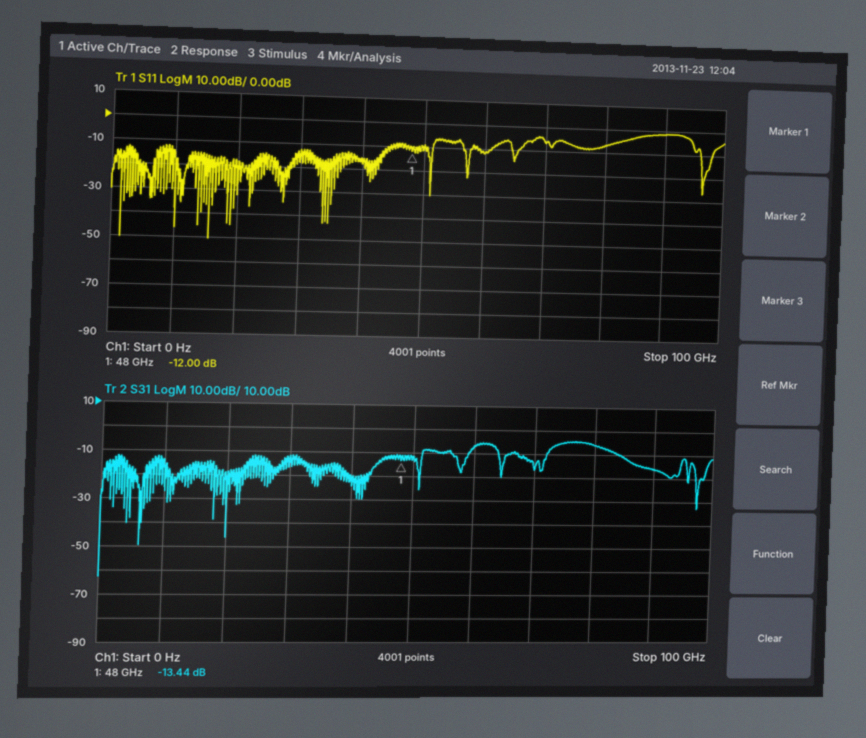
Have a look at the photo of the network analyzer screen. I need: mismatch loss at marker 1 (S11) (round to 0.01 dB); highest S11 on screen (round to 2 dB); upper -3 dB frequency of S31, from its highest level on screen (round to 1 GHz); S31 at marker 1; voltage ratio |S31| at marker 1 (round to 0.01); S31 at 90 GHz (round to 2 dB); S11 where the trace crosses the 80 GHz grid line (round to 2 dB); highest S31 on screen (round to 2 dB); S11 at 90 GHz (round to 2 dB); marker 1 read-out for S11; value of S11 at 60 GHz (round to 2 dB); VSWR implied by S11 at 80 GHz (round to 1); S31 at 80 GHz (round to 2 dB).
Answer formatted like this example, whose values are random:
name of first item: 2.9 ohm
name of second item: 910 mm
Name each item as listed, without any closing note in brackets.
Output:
mismatch loss at marker 1 (S11): 0.28 dB
highest S11 on screen: -2 dB
upper -3 dB frequency of S31, from its highest level on screen: 82 GHz
S31 at marker 1: -13.44 dB
voltage ratio |S31| at marker 1: 0.21
S31 at 90 GHz: -16 dB
S11 where the trace crosses the 80 GHz grid line: -6 dB
highest S31 on screen: -4 dB
S11 at 90 GHz: -2 dB
marker 1 read-out for S11: -12.00 dB
value of S11 at 60 GHz: -12 dB
VSWR implied by S11 at 80 GHz: 3
S31 at 80 GHz: -6 dB
